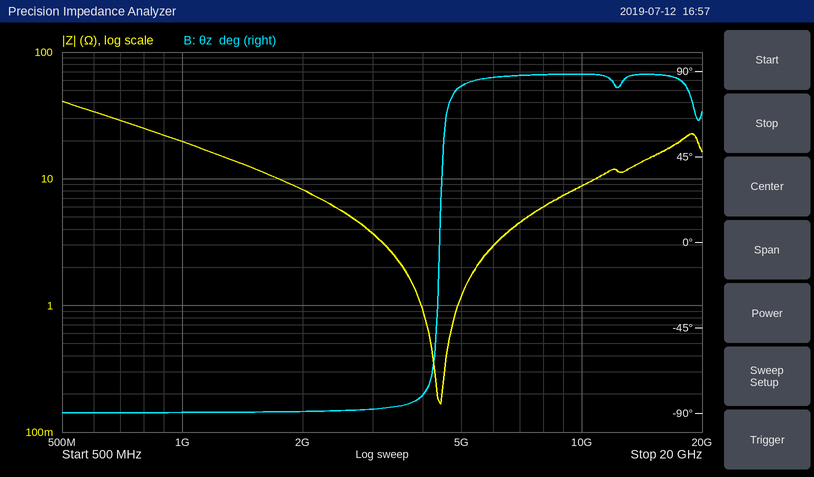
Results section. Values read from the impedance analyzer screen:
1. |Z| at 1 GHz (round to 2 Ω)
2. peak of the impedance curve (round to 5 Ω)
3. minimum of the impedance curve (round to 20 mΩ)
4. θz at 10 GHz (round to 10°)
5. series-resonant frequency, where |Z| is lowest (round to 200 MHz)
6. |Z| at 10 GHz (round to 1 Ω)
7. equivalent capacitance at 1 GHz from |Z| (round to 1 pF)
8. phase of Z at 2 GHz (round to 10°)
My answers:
20 Ω
40 Ω
160 mΩ
90°
4.4 GHz
9 Ω
8 pF
-90°
